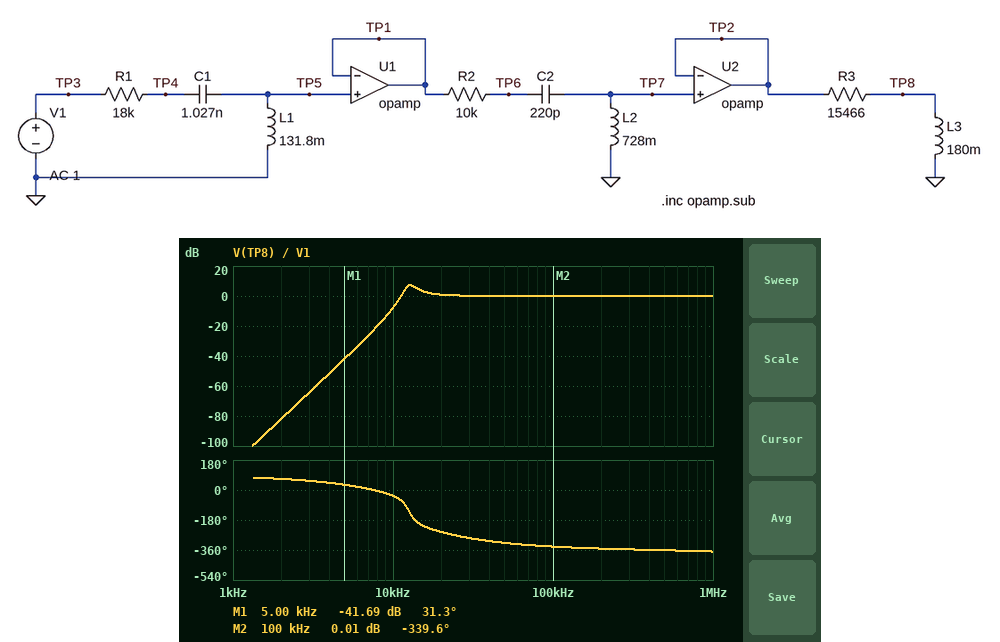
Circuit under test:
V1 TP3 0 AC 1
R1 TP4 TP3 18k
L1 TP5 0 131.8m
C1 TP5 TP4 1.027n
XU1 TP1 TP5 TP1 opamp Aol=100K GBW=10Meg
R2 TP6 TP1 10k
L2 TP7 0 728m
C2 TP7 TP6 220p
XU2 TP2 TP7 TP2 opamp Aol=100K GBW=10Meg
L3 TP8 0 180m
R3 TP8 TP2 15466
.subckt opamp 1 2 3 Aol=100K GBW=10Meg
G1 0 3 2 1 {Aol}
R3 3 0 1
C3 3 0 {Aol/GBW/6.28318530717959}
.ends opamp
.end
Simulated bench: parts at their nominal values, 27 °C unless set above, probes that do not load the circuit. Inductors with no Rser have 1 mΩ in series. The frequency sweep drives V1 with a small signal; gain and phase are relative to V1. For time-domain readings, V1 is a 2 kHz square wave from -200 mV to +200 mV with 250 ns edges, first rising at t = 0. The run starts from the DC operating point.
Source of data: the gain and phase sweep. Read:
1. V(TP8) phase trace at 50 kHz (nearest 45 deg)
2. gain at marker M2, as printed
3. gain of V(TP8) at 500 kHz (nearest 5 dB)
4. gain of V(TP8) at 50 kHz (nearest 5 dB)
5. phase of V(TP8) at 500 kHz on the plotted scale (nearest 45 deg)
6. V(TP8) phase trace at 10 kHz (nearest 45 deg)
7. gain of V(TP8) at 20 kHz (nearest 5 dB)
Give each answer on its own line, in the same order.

-315 deg
0.01 dB
0 dB
0 dB
-360 deg
-45 deg
0 dB
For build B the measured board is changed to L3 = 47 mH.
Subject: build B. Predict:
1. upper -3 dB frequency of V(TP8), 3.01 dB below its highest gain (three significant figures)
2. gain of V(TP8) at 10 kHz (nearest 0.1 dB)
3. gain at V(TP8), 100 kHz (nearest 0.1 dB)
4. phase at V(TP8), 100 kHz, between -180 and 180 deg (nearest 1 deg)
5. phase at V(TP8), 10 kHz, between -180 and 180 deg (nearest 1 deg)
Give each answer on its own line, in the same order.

6.51 MHz
-17.8 dB
-1.0 dB
40 deg
-10 deg
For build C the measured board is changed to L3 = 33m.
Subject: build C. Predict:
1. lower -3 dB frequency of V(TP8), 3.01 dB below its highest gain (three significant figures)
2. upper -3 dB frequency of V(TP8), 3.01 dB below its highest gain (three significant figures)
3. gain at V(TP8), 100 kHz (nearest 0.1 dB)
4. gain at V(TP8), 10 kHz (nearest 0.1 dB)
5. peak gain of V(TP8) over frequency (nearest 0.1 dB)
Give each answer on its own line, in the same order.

70.1 kHz
6.55 MHz
-1.8 dB
-20.8 dB
-0.1 dB
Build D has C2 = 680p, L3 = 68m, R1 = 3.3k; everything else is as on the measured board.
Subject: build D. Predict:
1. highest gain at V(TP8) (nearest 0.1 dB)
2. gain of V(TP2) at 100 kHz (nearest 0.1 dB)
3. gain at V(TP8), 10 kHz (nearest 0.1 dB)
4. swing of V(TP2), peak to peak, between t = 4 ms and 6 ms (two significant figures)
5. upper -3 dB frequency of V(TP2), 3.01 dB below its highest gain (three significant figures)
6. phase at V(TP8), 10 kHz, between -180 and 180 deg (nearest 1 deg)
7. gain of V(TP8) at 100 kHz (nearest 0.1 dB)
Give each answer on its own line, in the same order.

4.4 dB
0.2 dB
-5.7 dB
870 mV
16.2 kHz
-106 deg
-0.3 dB
